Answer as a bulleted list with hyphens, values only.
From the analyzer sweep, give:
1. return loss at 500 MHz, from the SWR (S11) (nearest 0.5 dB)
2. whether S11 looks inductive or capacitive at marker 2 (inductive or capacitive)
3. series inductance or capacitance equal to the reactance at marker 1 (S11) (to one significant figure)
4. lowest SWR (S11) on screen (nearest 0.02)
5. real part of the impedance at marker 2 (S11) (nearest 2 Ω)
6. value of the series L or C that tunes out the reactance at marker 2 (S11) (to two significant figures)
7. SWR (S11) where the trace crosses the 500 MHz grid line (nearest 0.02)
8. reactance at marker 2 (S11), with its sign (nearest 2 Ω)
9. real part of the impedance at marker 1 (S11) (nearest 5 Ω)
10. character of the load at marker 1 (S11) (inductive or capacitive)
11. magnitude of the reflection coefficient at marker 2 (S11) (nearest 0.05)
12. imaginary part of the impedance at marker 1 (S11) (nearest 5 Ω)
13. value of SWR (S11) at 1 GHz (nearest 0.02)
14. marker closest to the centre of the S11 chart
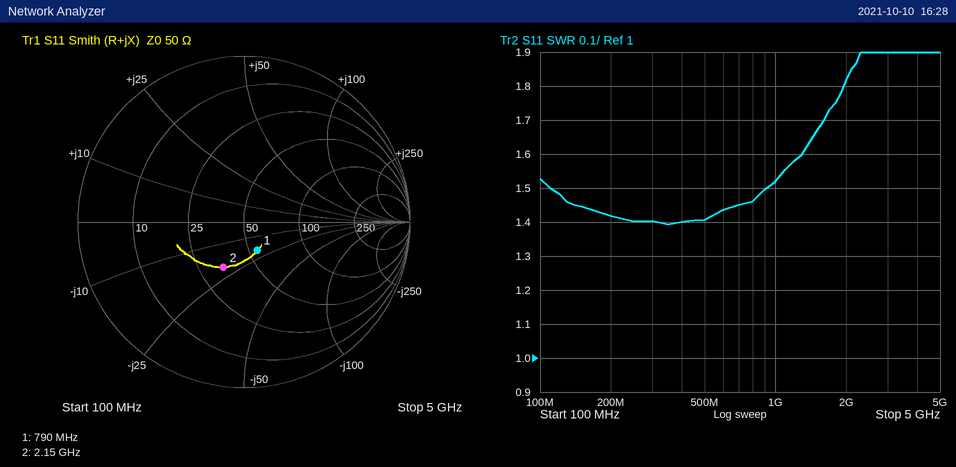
- 15.5 dB
- capacitive
- 10 pF
- 1.40
- 34 Ω
- 1.5 nH
- 1.40
- -20 Ω
- 55 Ω
- capacitive
- 0.30
- -20 Ω
- 1.52
- marker 1
